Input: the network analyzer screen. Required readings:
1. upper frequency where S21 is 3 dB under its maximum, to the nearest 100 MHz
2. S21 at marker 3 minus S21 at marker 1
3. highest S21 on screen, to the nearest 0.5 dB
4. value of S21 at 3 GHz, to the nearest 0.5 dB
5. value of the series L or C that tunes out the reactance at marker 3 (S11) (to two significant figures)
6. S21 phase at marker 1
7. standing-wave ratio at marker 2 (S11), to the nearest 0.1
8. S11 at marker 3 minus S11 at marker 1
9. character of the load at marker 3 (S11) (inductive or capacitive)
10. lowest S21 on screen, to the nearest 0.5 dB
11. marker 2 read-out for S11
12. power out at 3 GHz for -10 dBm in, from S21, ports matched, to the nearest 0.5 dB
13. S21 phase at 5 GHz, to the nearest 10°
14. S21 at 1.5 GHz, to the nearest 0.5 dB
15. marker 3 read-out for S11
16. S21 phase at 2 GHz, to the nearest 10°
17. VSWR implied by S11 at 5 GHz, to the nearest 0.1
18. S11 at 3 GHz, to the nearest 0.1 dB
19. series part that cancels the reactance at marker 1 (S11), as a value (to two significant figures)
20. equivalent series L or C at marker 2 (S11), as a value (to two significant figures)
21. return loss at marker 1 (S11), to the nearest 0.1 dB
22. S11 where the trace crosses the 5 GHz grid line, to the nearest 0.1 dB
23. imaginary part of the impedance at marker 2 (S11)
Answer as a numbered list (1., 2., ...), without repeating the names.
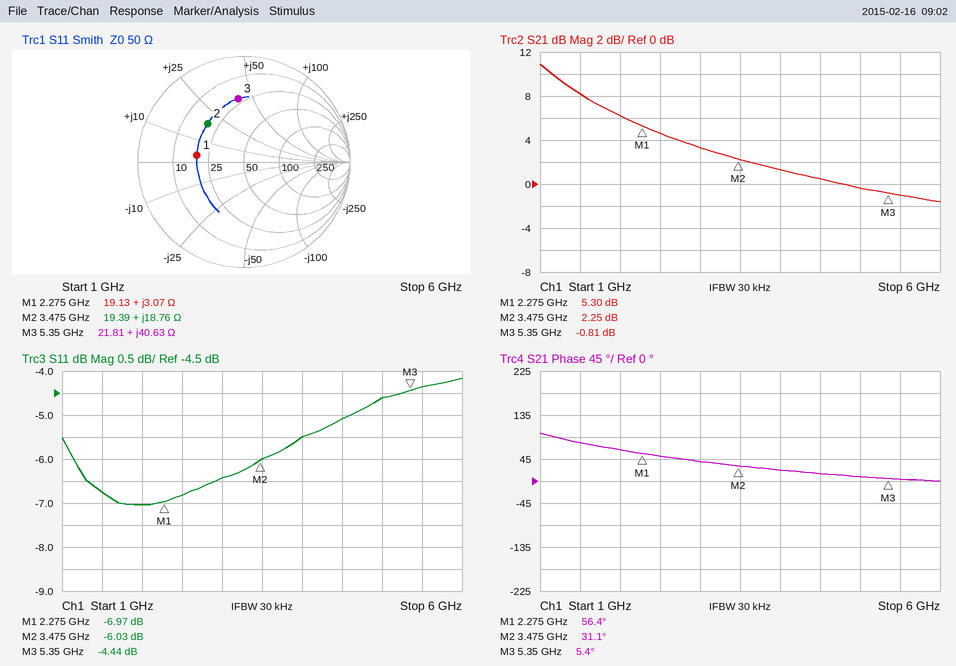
1. 1.6 GHz
2. -6.11 dB
3. 11.0 dB
4. 3.5 dB
5. 730 fF
6. 56.4°
7. 3.0
8. 2.53 dB
9. inductive
10. -1.5 dB
11. -6.03 dB
12. -6.5 dBm
13. 10°
14. 8.0 dB
15. -4.44 dB
16. 60°
17. 3.9
18. -6.4 dB
19. 23 pF
20. 860 pH
21. 7.0 dB
22. -4.6 dB
23. +18.76 Ω
